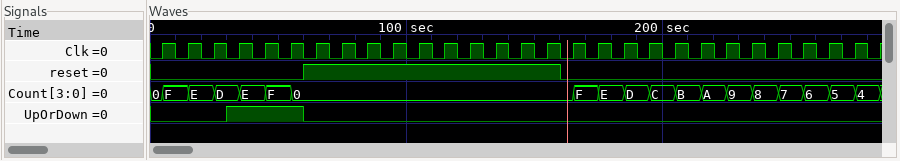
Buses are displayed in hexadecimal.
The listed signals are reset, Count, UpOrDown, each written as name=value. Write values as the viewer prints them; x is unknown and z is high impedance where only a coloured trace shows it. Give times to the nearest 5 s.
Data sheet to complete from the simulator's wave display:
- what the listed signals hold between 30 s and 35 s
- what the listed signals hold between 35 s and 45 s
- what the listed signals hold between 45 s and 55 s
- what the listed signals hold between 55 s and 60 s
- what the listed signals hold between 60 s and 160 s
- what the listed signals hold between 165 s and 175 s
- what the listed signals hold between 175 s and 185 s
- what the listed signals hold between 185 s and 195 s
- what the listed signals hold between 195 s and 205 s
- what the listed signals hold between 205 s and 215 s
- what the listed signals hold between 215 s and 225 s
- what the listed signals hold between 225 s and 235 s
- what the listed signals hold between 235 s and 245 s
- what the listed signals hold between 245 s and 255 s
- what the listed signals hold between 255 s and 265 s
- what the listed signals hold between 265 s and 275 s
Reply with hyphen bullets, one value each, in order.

- reset=0, Count=D, UpOrDown=1
- reset=0, Count=E, UpOrDown=1
- reset=0, Count=F, UpOrDown=1
- reset=0, Count=0, UpOrDown=1
- reset=1, Count=0, UpOrDown=0
- reset=0, Count=F, UpOrDown=0
- reset=0, Count=E, UpOrDown=0
- reset=0, Count=D, UpOrDown=0
- reset=0, Count=C, UpOrDown=0
- reset=0, Count=B, UpOrDown=0
- reset=0, Count=A, UpOrDown=0
- reset=0, Count=9, UpOrDown=0
- reset=0, Count=8, UpOrDown=0
- reset=0, Count=7, UpOrDown=0
- reset=0, Count=6, UpOrDown=0
- reset=0, Count=5, UpOrDown=0
